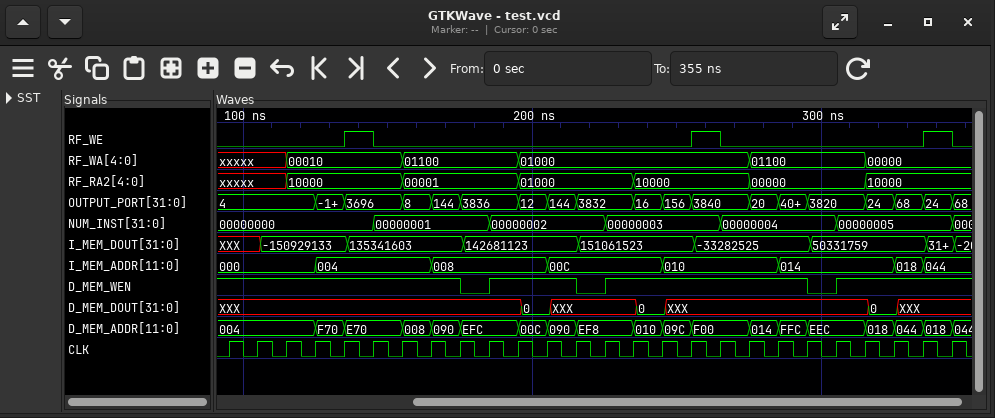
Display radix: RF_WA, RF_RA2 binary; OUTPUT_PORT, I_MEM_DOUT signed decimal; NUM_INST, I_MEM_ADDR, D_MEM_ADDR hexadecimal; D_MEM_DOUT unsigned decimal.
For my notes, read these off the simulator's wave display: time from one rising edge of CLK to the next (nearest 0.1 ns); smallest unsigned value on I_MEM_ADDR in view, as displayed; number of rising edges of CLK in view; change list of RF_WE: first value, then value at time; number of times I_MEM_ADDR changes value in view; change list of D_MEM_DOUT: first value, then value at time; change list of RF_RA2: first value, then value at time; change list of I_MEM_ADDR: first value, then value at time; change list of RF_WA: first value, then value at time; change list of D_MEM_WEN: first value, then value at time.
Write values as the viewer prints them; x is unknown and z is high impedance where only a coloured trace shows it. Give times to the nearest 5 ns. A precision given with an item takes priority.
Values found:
10 ns
000
26
0, 1 at 135 ns, 0 at 145 ns, 1 at 255 ns, 0 at 265 ns, 1 at 335 ns, 0 at 345 ns
7
XXX, 0 at 195 ns, XXX at 205 ns, 0 at 235 ns, XXX at 245 ns, 0 at 315 ns, XXX at 325 ns
xxxxx, 10000 at 115 ns, 00001 at 155 ns, 01000 at 195 ns, 10000 at 235 ns, 00000 at 275 ns, 10000 at 315 ns
000, 004 at 125 ns, 008 at 165 ns, 00C at 205 ns, 010 at 245 ns, 014 at 285 ns, 018 at 325 ns, 044 at 335 ns
xxxxx, 00010 at 115 ns, 01100 at 155 ns, 01000 at 195 ns, 01100 at 275 ns, 00000 at 315 ns
1, 0 at 175 ns, 1 at 185 ns, 0 at 215 ns, 1 at 225 ns, 0 at 295 ns, 1 at 305 ns
